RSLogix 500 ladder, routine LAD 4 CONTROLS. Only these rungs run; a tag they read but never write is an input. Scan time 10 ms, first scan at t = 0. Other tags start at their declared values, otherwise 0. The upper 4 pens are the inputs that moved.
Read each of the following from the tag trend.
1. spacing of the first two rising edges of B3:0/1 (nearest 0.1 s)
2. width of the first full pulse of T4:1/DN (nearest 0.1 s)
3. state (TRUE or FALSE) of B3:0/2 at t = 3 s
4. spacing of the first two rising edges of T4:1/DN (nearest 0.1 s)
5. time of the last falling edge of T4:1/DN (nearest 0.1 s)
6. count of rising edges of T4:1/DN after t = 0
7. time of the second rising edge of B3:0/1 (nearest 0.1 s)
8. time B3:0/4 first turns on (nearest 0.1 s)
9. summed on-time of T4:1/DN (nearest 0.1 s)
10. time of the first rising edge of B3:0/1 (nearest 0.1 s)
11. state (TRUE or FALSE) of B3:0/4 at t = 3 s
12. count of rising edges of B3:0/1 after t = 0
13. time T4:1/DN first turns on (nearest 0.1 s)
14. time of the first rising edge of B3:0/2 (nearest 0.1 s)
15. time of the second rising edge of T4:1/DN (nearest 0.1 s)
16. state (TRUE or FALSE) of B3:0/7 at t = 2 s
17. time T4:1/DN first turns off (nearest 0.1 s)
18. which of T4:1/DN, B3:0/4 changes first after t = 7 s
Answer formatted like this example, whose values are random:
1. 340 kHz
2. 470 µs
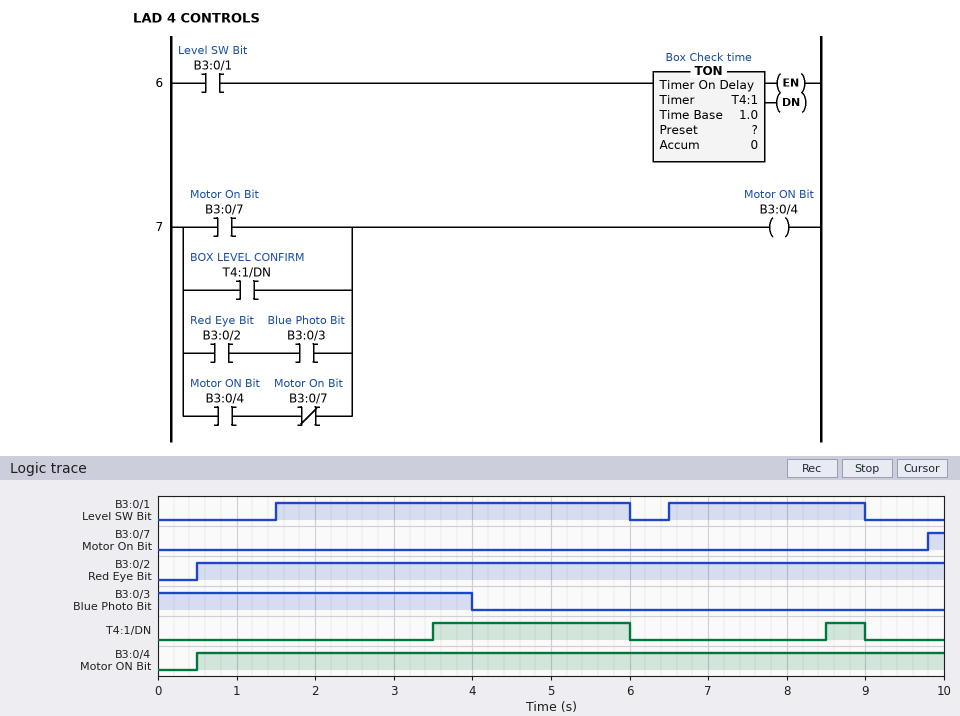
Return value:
1. 5.0 s
2. 2.5 s
3. TRUE
4. 5.0 s
5. 9.0 s
6. 2
7. 6.5 s
8. 0.5 s
9. 3.0 s
10. 1.5 s
11. TRUE
12. 2
13. 3.5 s
14. 0.5 s
15. 8.5 s
16. FALSE
17. 6.0 s
18. T4:1/DN
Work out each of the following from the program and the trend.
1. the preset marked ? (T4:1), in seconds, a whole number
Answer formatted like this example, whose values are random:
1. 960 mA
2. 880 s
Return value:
1. 2 s
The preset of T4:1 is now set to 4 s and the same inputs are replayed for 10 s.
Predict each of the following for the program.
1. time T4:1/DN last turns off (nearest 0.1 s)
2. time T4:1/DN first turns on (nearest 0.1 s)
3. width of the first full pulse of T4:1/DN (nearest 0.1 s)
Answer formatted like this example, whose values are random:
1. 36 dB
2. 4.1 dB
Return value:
1. 6.0 s
2. 5.5 s
3. 0.5 s
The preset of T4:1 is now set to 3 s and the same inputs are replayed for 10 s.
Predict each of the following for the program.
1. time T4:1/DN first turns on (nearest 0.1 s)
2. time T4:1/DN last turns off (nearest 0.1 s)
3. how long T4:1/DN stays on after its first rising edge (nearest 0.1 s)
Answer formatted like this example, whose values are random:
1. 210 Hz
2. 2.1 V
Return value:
1. 4.5 s
2. 6.0 s
3. 1.5 s
